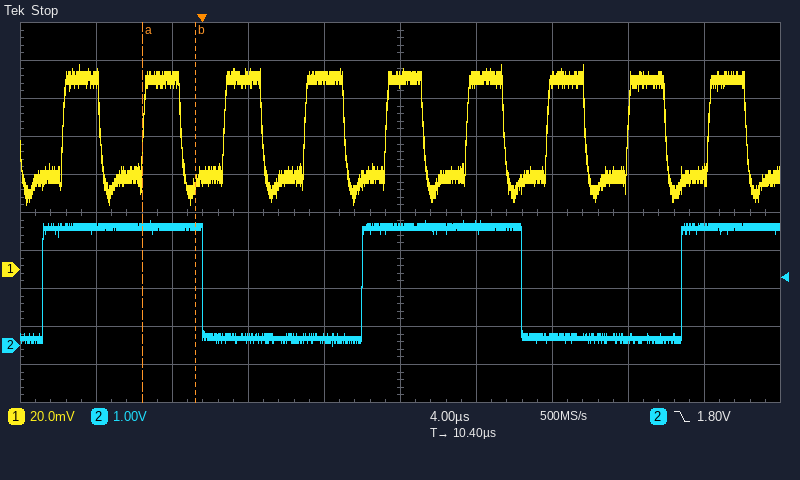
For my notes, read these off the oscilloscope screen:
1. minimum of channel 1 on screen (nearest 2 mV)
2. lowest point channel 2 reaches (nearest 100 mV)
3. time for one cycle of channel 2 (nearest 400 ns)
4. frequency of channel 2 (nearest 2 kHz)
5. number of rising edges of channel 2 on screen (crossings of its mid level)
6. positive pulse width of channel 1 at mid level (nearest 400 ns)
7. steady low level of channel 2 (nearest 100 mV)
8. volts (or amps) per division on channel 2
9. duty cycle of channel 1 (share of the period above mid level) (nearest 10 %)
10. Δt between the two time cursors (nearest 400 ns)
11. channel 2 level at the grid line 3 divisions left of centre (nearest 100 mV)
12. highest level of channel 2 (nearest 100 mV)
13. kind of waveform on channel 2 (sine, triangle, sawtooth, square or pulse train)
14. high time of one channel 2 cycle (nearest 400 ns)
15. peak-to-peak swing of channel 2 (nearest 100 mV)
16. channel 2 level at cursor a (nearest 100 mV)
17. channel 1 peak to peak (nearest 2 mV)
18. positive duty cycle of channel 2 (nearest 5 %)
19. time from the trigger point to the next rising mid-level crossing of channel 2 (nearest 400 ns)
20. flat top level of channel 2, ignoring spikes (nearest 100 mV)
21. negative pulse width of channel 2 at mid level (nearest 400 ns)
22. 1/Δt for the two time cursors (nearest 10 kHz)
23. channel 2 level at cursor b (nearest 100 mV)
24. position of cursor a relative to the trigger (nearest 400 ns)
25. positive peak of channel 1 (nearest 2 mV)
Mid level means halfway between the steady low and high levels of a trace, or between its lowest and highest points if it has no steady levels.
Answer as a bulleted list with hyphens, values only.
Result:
- 34 mV
- 0.0 V
- 16.8 µs
- 60 kHz
- 3
- 2.0 µs
- 200 mV
- 1 V
- 50 %
- 2.8 µs
- 3.1 V
- 3.3 V
- square
- 8.4 µs
- 3.3 V
- 3.1 V
- 74 mV
- 50 %
- 8.4 µs
- 3.1 V
- 8.4 µs
- 360 kHz
- 3.1 V
- -3.2 µs
- 108 mV
